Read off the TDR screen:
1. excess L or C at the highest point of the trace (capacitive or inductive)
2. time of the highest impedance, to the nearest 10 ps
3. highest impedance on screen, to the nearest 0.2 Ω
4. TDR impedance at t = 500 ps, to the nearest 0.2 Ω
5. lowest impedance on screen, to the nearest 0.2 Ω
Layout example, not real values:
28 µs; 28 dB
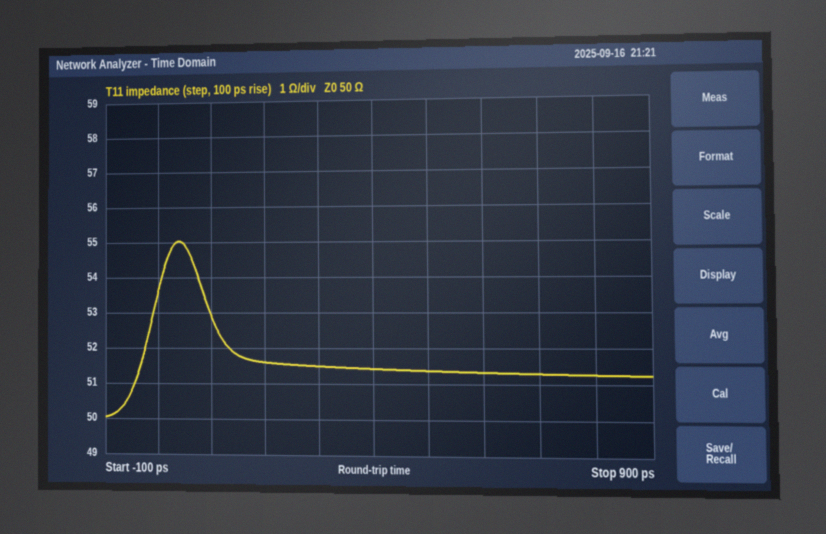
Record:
inductive; 40 ps; 55.0 Ω; 51.4 Ω; 50.0 Ω
